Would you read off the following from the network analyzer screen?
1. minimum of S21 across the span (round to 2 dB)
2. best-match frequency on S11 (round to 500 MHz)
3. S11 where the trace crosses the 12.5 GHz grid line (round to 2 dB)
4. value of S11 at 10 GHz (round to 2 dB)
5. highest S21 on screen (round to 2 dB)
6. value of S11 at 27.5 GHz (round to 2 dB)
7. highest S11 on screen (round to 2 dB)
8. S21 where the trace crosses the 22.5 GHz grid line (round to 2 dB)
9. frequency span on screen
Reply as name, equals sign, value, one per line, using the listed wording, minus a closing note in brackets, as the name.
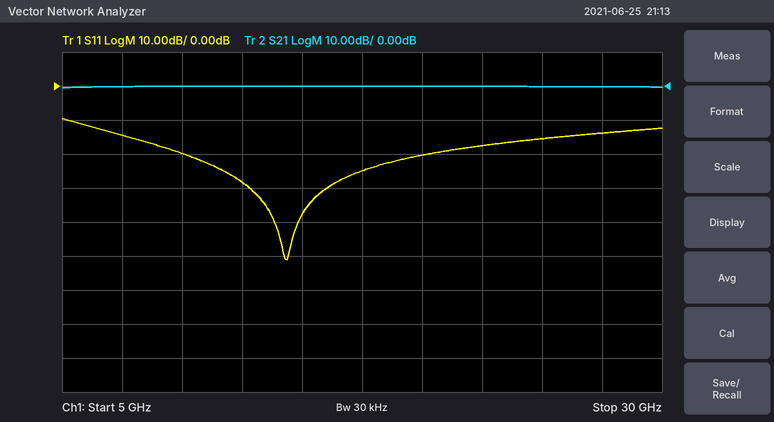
minimum of S21 across the span = 0 dB
best-match frequency on S11 = 14.5 GHz
S11 where the trace crosses the 12.5 GHz grid line = -28 dB
value of S11 at 10 GHz = -20 dB
highest S21 on screen = 0 dB
value of S11 at 27.5 GHz = -14 dB
highest S11 on screen = -10 dB
S21 where the trace crosses the 22.5 GHz grid line = 0 dB
frequency span on screen = 25 GHz
